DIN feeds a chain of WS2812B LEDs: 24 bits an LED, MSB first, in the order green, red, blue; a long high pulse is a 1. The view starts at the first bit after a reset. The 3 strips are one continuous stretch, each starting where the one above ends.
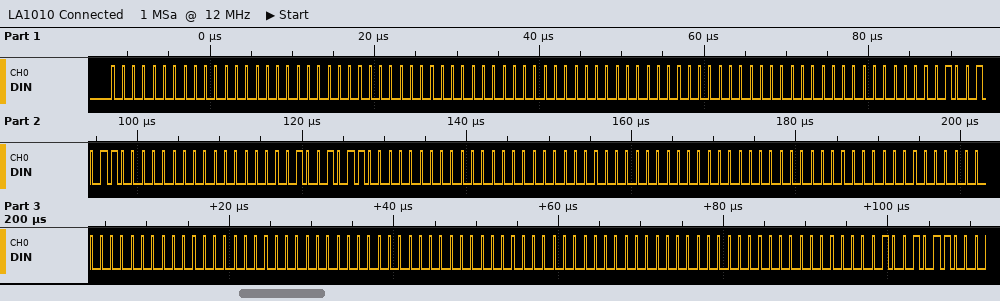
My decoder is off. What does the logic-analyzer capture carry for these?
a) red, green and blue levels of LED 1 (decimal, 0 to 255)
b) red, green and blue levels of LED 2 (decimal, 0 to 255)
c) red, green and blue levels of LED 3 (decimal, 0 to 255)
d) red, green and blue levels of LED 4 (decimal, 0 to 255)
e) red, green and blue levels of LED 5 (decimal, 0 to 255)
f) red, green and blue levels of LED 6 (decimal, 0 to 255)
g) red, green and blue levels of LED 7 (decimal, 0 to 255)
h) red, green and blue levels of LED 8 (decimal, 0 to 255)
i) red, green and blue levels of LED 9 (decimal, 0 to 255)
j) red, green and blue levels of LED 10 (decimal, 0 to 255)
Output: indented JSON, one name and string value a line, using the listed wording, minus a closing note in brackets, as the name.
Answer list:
{
  "red, green and blue levels of LED 1": "0, 0, 0",
  "red, green and blue levels of LED 2": "0, 0, 0",
  "red, green and blue levels of LED 3": "0, 0, 0",
  "red, green and blue levels of LED 4": "75, 0, 0",
  "red, green and blue levels of LED 5": "75, 0, 0",
  "red, green and blue levels of LED 6": "0, 0, 0",
  "red, green and blue levels of LED 7": "0, 0, 0",
  "red, green and blue levels of LED 8": "0, 0, 0",
  "red, green and blue levels of LED 9": "0, 0, 0",
  "red, green and blue levels of LED 10": "0, 0, 0"
}
